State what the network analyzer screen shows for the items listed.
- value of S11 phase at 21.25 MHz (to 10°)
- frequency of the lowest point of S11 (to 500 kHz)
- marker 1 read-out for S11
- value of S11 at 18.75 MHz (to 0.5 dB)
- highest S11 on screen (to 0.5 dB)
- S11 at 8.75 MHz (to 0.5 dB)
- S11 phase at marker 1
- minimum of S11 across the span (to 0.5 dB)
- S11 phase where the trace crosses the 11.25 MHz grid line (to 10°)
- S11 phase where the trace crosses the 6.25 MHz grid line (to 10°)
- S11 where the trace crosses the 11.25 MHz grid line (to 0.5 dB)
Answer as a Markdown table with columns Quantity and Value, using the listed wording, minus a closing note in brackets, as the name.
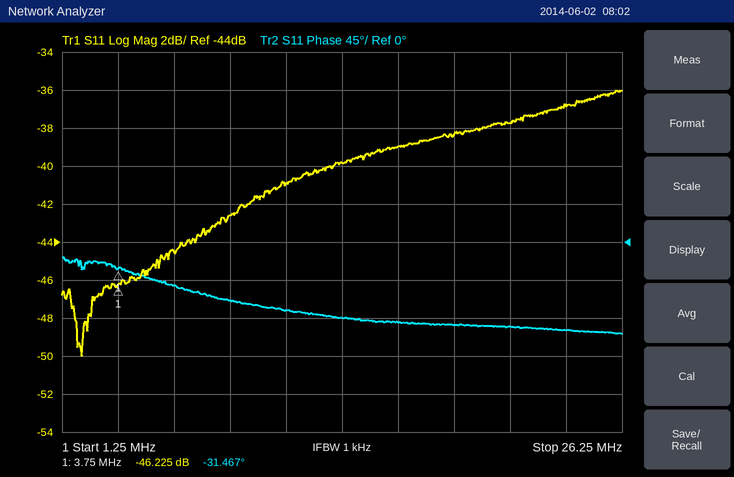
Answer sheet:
| Quantity | Value |
|---|---|
| value of S11 phase at 21.25 MHz | -100° |
| frequency of the lowest point of S11 | 2.0 MHz |
| marker 1 read-out for S11 | -46.225 dB |
| value of S11 at 18.75 MHz | -38.5 dB |
| highest S11 on screen | -36.0 dB |
| S11 at 8.75 MHz | -42.5 dB |
| S11 phase at marker 1 | -31.467° |
| minimum of S11 across the span | -50.0 dB |
| S11 phase where the trace crosses the 11.25 MHz grid line | -80° |
| S11 phase where the trace crosses the 6.25 MHz grid line | -50° |
| S11 where the trace crosses the 11.25 MHz grid line | -41.0 dB |
